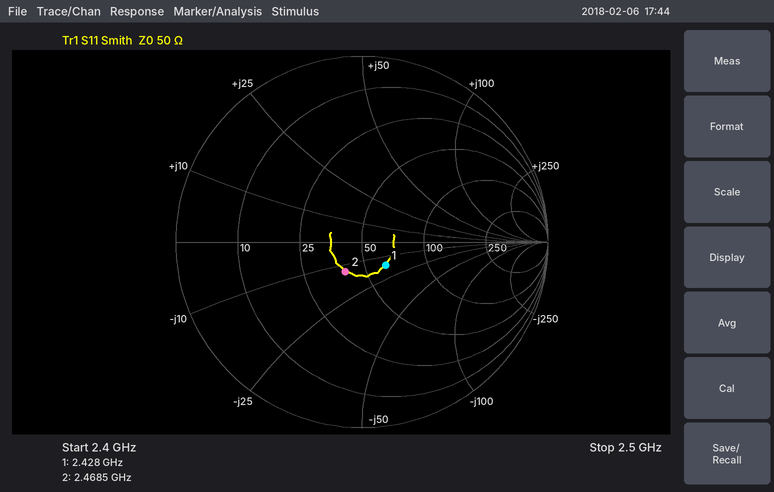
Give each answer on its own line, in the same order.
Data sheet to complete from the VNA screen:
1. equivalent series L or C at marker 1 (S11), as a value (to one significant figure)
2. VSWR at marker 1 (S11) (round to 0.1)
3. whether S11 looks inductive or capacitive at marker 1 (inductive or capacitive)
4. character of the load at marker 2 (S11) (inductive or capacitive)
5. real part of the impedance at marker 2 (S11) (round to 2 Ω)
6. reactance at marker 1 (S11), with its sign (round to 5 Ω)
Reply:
4 pF
1.4
capacitive
capacitive
40 Ω
-15 Ω
